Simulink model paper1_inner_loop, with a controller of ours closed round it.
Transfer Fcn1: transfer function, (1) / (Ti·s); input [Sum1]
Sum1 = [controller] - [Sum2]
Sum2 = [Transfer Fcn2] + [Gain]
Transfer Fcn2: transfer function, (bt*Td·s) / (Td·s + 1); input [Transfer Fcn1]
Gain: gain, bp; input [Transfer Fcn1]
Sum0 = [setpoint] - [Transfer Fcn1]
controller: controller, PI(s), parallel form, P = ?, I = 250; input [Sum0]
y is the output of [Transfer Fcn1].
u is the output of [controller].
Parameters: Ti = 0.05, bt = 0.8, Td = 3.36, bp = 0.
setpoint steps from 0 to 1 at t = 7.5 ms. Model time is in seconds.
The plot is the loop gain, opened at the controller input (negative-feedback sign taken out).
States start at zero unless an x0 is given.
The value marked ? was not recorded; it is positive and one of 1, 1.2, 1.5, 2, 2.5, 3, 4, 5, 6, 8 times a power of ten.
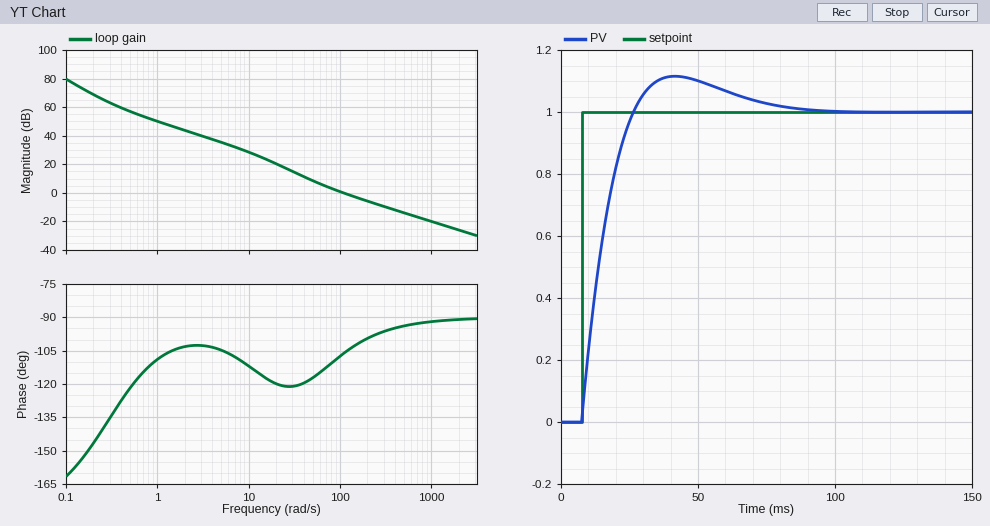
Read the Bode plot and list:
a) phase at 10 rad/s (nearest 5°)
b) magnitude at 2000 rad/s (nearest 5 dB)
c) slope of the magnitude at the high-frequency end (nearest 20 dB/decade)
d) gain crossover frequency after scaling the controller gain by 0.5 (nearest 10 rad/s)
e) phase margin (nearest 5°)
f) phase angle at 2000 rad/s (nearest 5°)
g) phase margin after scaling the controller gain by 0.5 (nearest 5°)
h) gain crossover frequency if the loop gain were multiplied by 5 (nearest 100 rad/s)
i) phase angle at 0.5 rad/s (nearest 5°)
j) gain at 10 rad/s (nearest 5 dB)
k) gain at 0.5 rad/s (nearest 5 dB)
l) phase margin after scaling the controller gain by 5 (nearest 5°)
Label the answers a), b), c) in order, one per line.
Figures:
a) -110°
b) -25 dB
c) -20 dB/decade
d) 60 rad/s
e) 75°
f) -90°
g) 65°
h) 500 rad/s
i) -120°
j) 30 dB
k) 55 dB
l) 85°
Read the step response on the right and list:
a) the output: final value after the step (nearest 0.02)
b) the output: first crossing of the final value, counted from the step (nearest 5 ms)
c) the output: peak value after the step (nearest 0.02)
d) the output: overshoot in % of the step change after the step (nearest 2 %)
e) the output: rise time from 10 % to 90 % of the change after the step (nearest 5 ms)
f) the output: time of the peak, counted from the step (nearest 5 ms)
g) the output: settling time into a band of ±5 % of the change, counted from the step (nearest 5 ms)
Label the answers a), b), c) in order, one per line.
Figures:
a) 1.00
b) 20 ms
c) 1.12
d) 12 %
e) 15 ms
f) 35 ms
g) 60 ms
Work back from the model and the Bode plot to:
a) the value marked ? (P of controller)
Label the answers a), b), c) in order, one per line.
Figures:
a) 5
